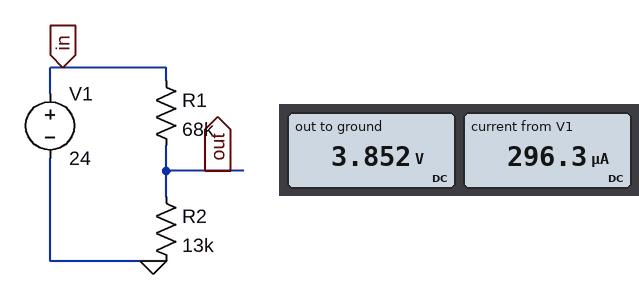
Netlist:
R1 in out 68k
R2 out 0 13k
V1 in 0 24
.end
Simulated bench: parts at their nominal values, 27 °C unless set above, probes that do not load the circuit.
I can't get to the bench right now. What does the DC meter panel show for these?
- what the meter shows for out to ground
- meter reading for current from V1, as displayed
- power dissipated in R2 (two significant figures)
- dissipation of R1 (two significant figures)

3.852 V
296.3 µA
1.1 mW
6.0 mW
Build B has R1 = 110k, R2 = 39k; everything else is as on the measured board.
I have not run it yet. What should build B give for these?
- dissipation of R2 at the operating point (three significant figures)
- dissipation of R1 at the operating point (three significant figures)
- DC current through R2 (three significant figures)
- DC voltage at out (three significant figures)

1.01 mW
2.85 mW
161 µA
6.28 V
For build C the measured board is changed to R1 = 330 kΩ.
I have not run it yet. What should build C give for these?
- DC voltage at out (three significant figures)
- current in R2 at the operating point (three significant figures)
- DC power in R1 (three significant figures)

910 mV
70.0 µA
1.62 mW
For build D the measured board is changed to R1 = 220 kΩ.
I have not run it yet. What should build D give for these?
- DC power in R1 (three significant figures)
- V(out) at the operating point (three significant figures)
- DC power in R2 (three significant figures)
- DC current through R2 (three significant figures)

2.33 mW
1.34 V
138 µW
103 µA
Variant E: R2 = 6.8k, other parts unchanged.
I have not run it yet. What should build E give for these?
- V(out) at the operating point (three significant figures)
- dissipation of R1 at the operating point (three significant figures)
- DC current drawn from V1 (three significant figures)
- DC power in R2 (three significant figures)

2.18 V
7.00 mW
321 µA
700 µW
